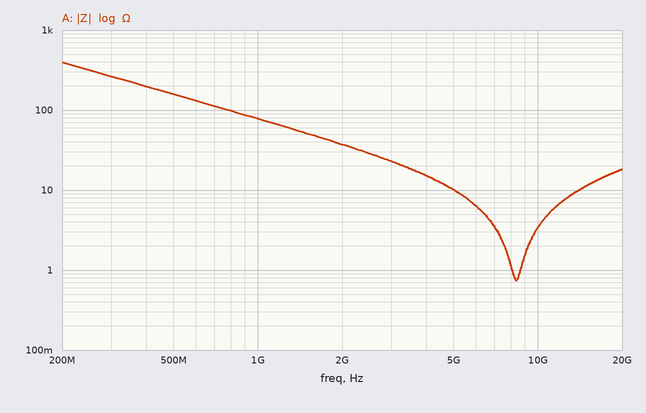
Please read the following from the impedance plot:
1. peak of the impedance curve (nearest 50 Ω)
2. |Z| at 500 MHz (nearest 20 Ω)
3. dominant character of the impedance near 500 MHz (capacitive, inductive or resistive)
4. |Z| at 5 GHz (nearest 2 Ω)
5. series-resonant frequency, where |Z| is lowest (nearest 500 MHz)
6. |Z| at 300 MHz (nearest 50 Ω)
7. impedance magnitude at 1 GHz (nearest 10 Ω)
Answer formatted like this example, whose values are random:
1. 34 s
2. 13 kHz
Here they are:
1. 400 Ω
2. 160 Ω
3. capacitive
4. 10 Ω
5. 8.5 GHz
6. 250 Ω
7. 80 Ω
